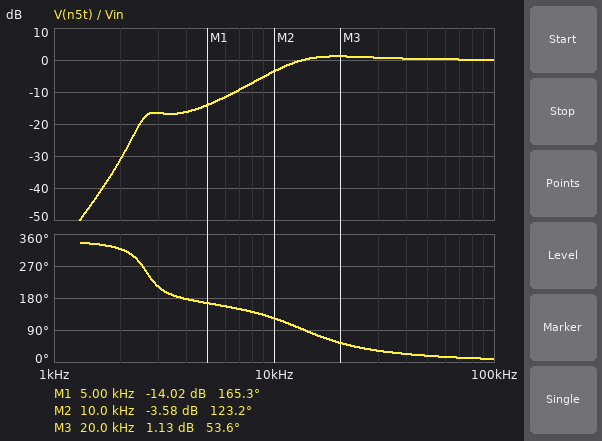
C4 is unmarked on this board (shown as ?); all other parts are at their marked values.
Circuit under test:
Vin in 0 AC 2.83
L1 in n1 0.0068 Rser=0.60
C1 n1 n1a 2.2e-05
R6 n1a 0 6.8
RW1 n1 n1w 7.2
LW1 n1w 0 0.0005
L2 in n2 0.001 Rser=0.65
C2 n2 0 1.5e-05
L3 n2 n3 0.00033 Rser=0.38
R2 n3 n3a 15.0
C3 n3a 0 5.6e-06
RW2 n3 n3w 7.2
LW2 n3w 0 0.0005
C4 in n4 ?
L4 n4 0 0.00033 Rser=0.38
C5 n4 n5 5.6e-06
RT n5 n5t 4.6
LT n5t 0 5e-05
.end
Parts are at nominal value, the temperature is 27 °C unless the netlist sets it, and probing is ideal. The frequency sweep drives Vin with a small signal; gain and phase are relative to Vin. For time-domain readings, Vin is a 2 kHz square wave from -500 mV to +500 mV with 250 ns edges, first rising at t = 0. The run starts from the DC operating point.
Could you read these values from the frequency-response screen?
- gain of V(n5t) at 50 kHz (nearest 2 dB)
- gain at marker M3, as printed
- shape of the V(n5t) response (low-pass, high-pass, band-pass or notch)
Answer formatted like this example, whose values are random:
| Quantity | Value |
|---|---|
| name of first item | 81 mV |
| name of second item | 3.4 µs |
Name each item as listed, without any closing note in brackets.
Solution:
| Quantity | Value |
|---|---|
| gain of V(n5t) at 50 kHz | 0 dB |
| gain at marker M3, as printed | 1.13 dB |
| shape of the V(n5t) response | high-pass |
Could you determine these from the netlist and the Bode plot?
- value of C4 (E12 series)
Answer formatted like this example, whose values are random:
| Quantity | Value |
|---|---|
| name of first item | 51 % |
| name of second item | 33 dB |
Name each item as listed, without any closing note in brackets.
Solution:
| Quantity | Value |
|---|---|
| value of C4 | 5.6 µF |
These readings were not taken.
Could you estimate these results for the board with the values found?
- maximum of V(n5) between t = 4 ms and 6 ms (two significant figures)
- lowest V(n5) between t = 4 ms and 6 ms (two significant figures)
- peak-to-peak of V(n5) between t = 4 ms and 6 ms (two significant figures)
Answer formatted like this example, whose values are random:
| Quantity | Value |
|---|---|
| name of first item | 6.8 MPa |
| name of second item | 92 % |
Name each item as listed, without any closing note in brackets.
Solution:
| Quantity | Value |
|---|---|
| maximum of V(n5) between t = 4 ms and 6 ms | 850 mV |
| lowest V(n5) between t = 4 ms and 6 ms | -850 mV |
| peak-to-peak of V(n5) between t = 4 ms and 6 ms | 1.7 V |
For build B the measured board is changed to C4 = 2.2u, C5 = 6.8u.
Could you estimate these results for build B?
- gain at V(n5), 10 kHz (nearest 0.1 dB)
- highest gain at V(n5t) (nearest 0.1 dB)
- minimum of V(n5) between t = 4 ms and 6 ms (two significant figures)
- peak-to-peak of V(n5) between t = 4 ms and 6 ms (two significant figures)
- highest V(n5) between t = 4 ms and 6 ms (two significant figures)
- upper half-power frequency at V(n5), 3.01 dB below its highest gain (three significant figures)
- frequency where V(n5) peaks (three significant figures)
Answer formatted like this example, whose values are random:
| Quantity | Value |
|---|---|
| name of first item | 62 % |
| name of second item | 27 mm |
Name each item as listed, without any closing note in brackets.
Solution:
| Quantity | Value |
|---|---|
| gain at V(n5), 10 kHz | -2.4 dB |
| highest gain at V(n5t) | 3.3 dB |
| minimum of V(n5) between t = 4 ms and 6 ms | -960 mV |
| peak-to-peak of V(n5) between t = 4 ms and 6 ms | 1.9 V |
| highest V(n5) between t = 4 ms and 6 ms | 960 mV |
| upper half-power frequency at V(n5), 3.01 dB below its highest gain | 36.8 kHz |
| frequency where V(n5) peaks | 19.4 kHz |
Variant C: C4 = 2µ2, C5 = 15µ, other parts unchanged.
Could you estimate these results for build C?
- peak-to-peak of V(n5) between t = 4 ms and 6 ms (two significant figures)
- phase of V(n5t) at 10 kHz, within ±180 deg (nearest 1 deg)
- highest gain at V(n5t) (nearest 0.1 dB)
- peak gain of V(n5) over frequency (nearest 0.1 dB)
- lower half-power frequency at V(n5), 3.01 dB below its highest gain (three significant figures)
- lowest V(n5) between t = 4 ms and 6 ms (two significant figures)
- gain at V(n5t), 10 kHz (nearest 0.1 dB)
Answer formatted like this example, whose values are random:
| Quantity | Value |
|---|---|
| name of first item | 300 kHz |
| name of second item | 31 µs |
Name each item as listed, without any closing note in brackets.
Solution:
| Quantity | Value |
|---|---|
| peak-to-peak of V(n5) between t = 4 ms and 6 ms | 2.0 V |
| phase of V(n5t) at 10 kHz, within ±180 deg | 153 deg |
| highest gain at V(n5t) | 2.9 dB |
| peak gain of V(n5) over frequency | 4.9 dB |
| lower half-power frequency at V(n5), 3.01 dB below its highest gain | 12.6 kHz |
| lowest V(n5) between t = 4 ms and 6 ms | -980 mV |
| gain at V(n5t), 10 kHz | -6.5 dB |
